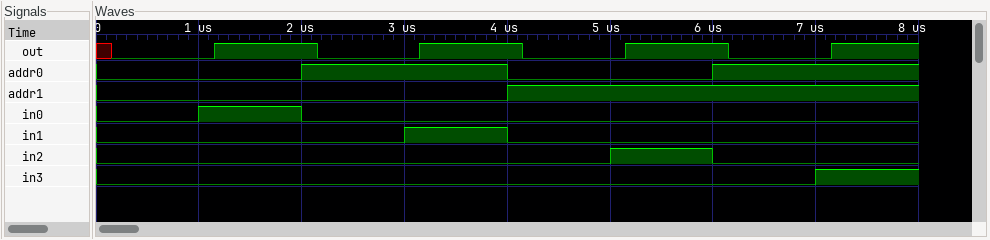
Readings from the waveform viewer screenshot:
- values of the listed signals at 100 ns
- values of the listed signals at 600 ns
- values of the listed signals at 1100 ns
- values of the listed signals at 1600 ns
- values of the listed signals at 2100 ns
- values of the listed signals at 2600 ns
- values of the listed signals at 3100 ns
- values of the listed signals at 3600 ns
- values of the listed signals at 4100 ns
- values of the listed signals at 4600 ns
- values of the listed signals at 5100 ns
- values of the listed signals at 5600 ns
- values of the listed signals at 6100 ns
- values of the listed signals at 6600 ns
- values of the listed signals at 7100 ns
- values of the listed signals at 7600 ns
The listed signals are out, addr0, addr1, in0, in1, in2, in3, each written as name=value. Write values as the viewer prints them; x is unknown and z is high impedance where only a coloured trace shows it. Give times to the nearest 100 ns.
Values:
out=x, addr0=0, addr1=0, in0=0, in1=0, in2=0, in3=0
out=0, addr0=0, addr1=0, in0=0, in1=0, in2=0, in3=0
out=0, addr0=0, addr1=0, in0=1, in1=0, in2=0, in3=0
out=1, addr0=0, addr1=0, in0=1, in1=0, in2=0, in3=0
out=1, addr0=1, addr1=0, in0=0, in1=0, in2=0, in3=0
out=0, addr0=1, addr1=0, in0=0, in1=0, in2=0, in3=0
out=0, addr0=1, addr1=0, in0=0, in1=1, in2=0, in3=0
out=1, addr0=1, addr1=0, in0=0, in1=1, in2=0, in3=0
out=1, addr0=0, addr1=1, in0=0, in1=0, in2=0, in3=0
out=0, addr0=0, addr1=1, in0=0, in1=0, in2=0, in3=0
out=0, addr0=0, addr1=1, in0=0, in1=0, in2=1, in3=0
out=1, addr0=0, addr1=1, in0=0, in1=0, in2=1, in3=0
out=1, addr0=1, addr1=1, in0=0, in1=0, in2=0, in3=0
out=0, addr0=1, addr1=1, in0=0, in1=0, in2=0, in3=0
out=0, addr0=1, addr1=1, in0=0, in1=0, in2=0, in3=1
out=1, addr0=1, addr1=1, in0=0, in1=0, in2=0, in3=1
